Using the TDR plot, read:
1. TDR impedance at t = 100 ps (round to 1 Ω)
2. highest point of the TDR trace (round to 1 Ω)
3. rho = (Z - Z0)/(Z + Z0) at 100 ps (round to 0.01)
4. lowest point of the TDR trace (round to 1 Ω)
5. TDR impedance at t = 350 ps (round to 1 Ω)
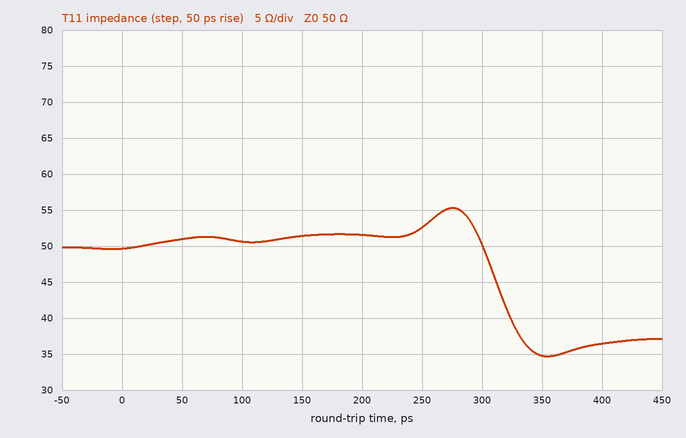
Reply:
51 Ω
55 Ω
+0.01
35 Ω
35 Ω
